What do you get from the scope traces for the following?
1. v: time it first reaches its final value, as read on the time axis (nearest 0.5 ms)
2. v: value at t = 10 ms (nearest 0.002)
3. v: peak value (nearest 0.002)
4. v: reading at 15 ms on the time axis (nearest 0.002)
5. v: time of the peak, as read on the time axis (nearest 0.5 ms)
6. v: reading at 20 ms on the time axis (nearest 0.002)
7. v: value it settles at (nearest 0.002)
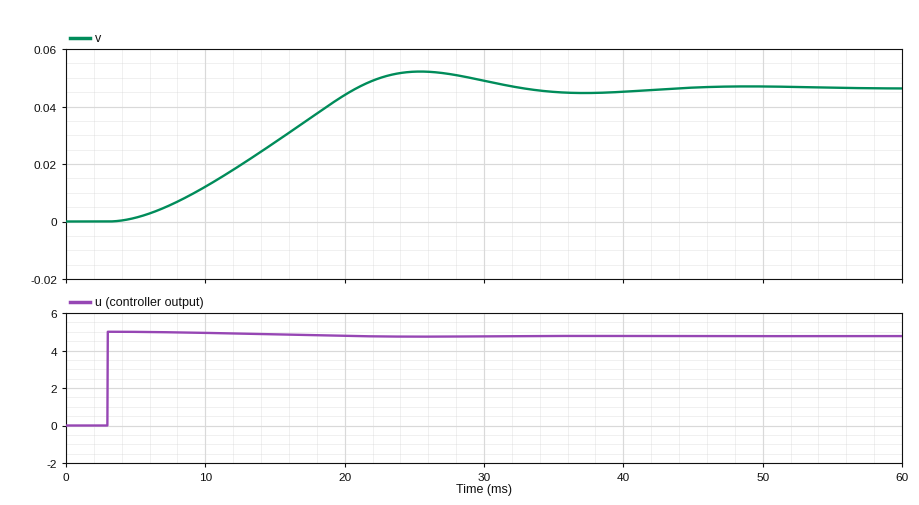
21.0 ms
0.012
0.052
0.028
25.5 ms
0.044
0.046
